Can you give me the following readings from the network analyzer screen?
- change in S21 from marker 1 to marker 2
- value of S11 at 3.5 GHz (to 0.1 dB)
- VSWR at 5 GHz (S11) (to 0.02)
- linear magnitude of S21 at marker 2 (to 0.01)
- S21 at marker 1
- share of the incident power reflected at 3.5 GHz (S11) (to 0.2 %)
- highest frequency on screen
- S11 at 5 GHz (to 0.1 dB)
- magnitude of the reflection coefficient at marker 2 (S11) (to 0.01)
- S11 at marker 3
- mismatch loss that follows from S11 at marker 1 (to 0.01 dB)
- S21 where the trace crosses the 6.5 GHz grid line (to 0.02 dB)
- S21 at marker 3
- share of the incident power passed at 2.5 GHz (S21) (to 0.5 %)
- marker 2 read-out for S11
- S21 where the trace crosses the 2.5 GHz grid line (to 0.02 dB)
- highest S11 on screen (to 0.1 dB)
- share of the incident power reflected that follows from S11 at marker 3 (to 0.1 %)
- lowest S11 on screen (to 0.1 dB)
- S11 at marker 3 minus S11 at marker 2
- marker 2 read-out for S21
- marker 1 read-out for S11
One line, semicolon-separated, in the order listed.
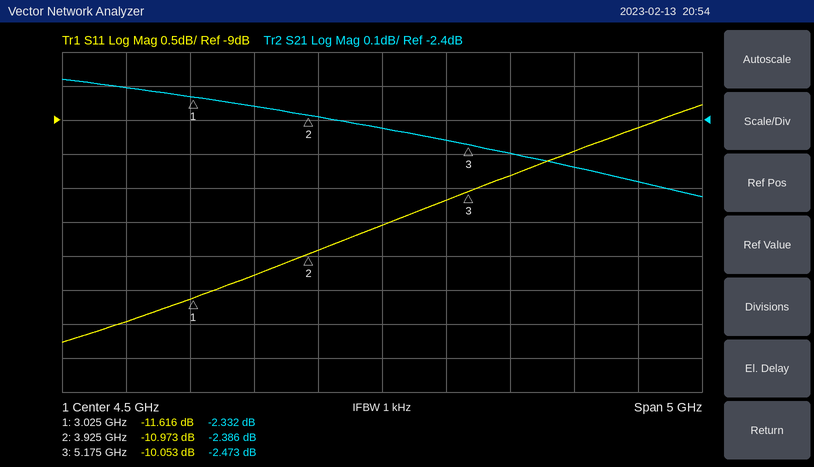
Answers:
-0.054 dB; -11.3 dB; 1.90; 0.76; -2.332 dB; 7.4 %; 7 GHz; -10.2 dB; 0.28; -10.053 dB; 0.31 dB; -2.58 dB; -2.473 dB; 59.0 %; -10.973 dB; -2.30 dB; -8.8 dB; 9.9 %; -12.3 dB; 0.920 dB; -2.386 dB; -11.616 dB
